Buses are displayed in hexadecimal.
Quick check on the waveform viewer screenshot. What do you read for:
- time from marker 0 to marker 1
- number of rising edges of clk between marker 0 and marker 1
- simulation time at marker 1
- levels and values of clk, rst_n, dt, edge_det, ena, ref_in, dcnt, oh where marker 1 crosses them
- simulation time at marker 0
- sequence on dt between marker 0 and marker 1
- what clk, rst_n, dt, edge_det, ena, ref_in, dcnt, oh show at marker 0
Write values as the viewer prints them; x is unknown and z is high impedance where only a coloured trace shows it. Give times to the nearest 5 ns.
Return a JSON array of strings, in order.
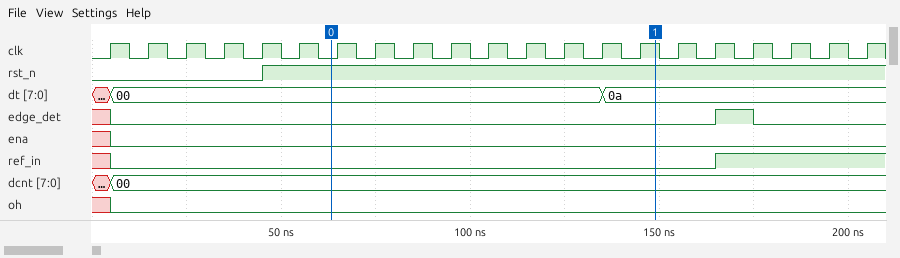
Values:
["85 ns", "9", "150 ns", "clk=1, rst_n=1, dt=0a, edge_det=0, ena=0, ref_in=0, dcnt=00, oh=0", "65 ns", "00, 0a", "clk=0, rst_n=1, dt=00, edge_det=0, ena=0, ref_in=0, dcnt=00, oh=0"]
